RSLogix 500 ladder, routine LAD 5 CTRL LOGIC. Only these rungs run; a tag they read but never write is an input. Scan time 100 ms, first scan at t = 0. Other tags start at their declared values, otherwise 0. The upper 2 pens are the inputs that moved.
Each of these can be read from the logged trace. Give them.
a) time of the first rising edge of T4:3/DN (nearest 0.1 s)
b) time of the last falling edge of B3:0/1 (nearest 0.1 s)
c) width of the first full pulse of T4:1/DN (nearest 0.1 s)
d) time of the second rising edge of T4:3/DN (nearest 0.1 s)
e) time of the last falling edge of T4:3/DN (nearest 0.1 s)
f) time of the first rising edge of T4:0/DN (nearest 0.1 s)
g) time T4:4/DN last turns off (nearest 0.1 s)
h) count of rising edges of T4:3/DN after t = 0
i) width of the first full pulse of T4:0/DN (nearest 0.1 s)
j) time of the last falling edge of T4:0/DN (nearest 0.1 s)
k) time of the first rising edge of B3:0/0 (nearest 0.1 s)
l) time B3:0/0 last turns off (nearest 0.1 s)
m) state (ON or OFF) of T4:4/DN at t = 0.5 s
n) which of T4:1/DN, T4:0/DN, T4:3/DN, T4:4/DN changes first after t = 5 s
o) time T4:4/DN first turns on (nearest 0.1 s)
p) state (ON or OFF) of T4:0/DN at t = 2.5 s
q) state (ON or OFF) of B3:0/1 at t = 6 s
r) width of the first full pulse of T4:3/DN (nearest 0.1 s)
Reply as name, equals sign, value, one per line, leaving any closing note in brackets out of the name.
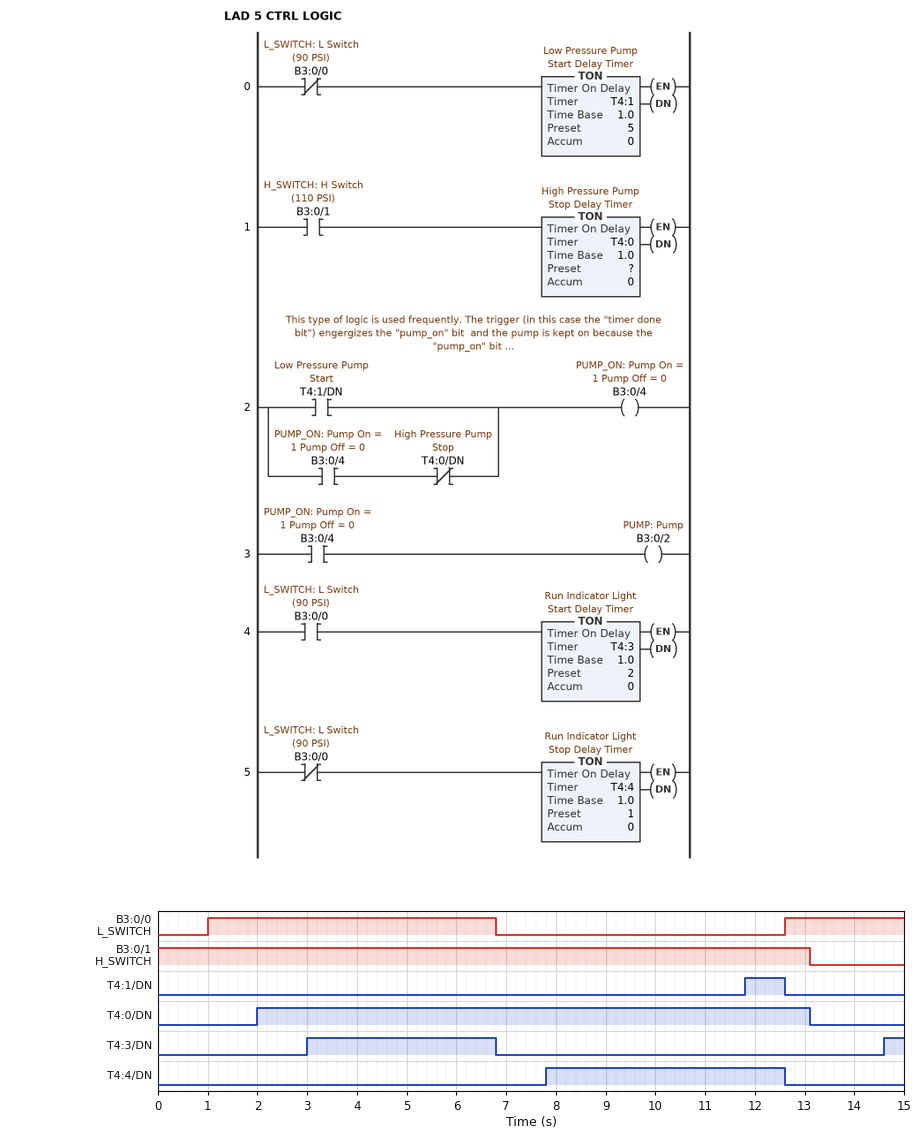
time of the first rising edge of T4:3/DN = 3.0 s
time of the last falling edge of B3:0/1 = 13.1 s
width of the first full pulse of T4:1/DN = 0.8 s
time of the second rising edge of T4:3/DN = 14.6 s
time of the last falling edge of T4:3/DN = 6.8 s
time of the first rising edge of T4:0/DN = 2.0 s
time T4:4/DN last turns off = 12.6 s
count of rising edges of T4:3/DN after t = 0 = 2
width of the first full pulse of T4:0/DN = 11.1 s
time of the last falling edge of T4:0/DN = 13.1 s
time of the first rising edge of B3:0/0 = 1.0 s
time B3:0/0 last turns off = 6.8 s
state (ON or OFF) of T4:4/DN at t = 0.5 s = OFF
which of T4:1/DN, T4:0/DN, T4:3/DN, T4:4/DN changes first after t = 5 s = T4:3/DN
time T4:4/DN first turns on = 7.8 s
state (ON or OFF) of T4:0/DN at t = 2.5 s = ON
state (ON or OFF) of B3:0/1 at t = 6 s = ON
width of the first full pulse of T4:3/DN = 3.8 s
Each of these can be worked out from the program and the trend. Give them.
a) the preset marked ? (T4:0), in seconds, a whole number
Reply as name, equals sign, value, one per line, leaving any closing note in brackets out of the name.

the preset marked ? (T4:0), in seconds, a whole number = 2 s
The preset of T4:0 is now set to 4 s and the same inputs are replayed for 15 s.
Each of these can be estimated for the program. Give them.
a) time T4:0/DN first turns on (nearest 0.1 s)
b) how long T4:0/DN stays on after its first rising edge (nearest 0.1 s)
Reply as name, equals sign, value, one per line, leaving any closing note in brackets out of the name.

time T4:0/DN first turns on = 4.0 s
how long T4:0/DN stays on after its first rising edge = 9.1 s
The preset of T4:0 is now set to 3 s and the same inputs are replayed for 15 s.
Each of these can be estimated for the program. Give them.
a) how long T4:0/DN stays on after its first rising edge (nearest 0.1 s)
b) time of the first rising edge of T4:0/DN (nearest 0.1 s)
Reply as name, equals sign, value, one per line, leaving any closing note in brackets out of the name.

how long T4:0/DN stays on after its first rising edge = 10.1 s
time of the first rising edge of T4:0/DN = 3.0 s
